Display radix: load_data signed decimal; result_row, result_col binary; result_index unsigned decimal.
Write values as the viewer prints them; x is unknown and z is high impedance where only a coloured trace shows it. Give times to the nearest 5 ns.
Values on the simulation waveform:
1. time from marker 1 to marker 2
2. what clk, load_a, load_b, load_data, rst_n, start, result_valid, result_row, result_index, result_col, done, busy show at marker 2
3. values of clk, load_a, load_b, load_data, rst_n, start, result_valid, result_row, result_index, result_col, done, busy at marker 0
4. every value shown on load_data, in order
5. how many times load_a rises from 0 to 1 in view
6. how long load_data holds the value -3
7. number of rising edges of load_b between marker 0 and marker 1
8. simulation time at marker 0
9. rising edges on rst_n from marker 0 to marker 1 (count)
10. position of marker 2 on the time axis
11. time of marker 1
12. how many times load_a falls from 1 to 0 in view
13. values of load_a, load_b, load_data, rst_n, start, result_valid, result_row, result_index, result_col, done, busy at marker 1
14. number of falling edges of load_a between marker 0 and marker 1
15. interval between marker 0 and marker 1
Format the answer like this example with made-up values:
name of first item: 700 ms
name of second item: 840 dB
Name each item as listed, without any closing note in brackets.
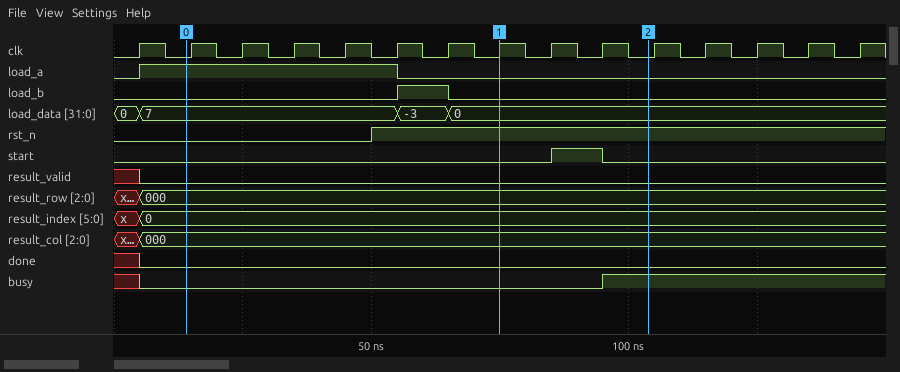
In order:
time from marker 1 to marker 2: 30 ns
what clk, load_a, load_b, load_data, rst_n, start, result_valid, result_row, result_index, result_col, done, busy show at marker 2: clk=0, load_a=0, load_b=0, load_data=0, rst_n=1, start=0, result_valid=0, result_row=000, result_index=0, result_col=000, done=0, busy=1
values of clk, load_a, load_b, load_data, rst_n, start, result_valid, result_row, result_index, result_col, done, busy at marker 0: clk=0, load_a=1, load_b=0, load_data=7, rst_n=0, start=0, result_valid=0, result_row=000, result_index=0, result_col=000, done=0, busy=0
every value shown on load_data, in order: 0, 7, -3, 0
how many times load_a rises from 0 to 1 in view: 1
how long load_data holds the value -3: 10 ns
number of rising edges of load_b between marker 0 and marker 1: 1
simulation time at marker 0: 15 ns
rising edges on rst_n from marker 0 to marker 1: 1
position of marker 2 on the time axis: 105 ns
time of marker 1: 75 ns
how many times load_a falls from 1 to 0 in view: 1
values of load_a, load_b, load_data, rst_n, start, result_valid, result_row, result_index, result_col, done, busy at marker 1: load_a=0, load_b=0, load_data=0, rst_n=1, start=0, result_valid=0, result_row=000, result_index=0, result_col=000, done=0, busy=0
number of falling edges of load_a between marker 0 and marker 1: 1
interval between marker 0 and marker 1: 60 ns
